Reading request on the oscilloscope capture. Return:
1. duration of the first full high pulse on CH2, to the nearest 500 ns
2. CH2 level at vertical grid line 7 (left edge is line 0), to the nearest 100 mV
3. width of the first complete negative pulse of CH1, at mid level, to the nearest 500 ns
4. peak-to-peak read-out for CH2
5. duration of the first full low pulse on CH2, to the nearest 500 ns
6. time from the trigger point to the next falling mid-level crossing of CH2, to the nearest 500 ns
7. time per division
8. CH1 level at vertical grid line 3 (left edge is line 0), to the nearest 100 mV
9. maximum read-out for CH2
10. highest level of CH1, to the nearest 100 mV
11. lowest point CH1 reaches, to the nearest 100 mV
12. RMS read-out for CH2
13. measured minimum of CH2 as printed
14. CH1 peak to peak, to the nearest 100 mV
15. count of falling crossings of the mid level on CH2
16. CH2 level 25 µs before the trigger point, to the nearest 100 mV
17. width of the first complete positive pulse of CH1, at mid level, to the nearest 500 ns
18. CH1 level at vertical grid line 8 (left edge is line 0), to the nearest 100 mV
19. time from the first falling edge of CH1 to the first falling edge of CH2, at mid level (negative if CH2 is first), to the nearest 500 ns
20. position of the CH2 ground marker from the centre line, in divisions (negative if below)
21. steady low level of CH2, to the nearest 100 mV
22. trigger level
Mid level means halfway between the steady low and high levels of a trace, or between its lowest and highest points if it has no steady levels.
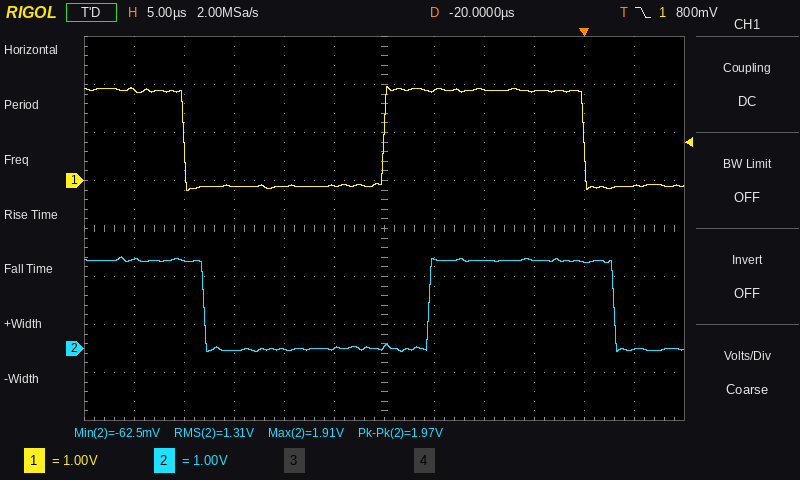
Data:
18.5 µs
1.8 V
20.0 µs
1.97 V
22.5 µs
3.0 µs
5 µs
-100 mV
1.91 V
2.0 V
-200 mV
1.31 V
-62.5 mV
2.2 V
2
0.0 V
20.0 µs
1.9 V
+2.0 µs
-2.5 div
0.0 V
800 mV
